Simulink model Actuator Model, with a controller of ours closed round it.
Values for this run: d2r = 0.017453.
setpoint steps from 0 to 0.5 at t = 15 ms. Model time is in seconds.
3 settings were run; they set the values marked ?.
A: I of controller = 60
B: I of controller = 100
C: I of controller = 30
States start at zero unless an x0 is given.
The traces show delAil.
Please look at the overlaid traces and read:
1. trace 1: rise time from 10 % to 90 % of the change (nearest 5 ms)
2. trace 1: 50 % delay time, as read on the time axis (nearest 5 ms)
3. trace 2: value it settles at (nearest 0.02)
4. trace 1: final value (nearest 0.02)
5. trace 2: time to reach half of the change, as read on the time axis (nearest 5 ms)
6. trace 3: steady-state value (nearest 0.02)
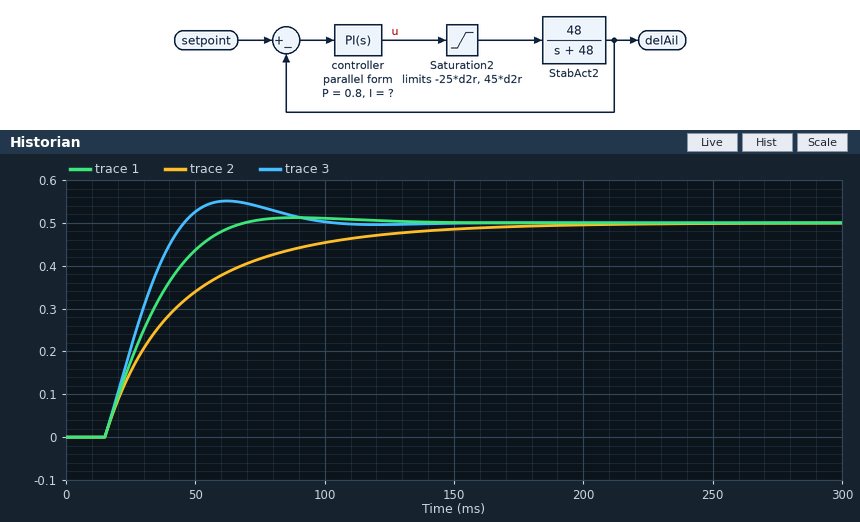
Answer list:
35 ms
30 ms
0.50
0.50
35 ms
0.50
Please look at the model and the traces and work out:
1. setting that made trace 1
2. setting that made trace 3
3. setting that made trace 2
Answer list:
A
B
C
